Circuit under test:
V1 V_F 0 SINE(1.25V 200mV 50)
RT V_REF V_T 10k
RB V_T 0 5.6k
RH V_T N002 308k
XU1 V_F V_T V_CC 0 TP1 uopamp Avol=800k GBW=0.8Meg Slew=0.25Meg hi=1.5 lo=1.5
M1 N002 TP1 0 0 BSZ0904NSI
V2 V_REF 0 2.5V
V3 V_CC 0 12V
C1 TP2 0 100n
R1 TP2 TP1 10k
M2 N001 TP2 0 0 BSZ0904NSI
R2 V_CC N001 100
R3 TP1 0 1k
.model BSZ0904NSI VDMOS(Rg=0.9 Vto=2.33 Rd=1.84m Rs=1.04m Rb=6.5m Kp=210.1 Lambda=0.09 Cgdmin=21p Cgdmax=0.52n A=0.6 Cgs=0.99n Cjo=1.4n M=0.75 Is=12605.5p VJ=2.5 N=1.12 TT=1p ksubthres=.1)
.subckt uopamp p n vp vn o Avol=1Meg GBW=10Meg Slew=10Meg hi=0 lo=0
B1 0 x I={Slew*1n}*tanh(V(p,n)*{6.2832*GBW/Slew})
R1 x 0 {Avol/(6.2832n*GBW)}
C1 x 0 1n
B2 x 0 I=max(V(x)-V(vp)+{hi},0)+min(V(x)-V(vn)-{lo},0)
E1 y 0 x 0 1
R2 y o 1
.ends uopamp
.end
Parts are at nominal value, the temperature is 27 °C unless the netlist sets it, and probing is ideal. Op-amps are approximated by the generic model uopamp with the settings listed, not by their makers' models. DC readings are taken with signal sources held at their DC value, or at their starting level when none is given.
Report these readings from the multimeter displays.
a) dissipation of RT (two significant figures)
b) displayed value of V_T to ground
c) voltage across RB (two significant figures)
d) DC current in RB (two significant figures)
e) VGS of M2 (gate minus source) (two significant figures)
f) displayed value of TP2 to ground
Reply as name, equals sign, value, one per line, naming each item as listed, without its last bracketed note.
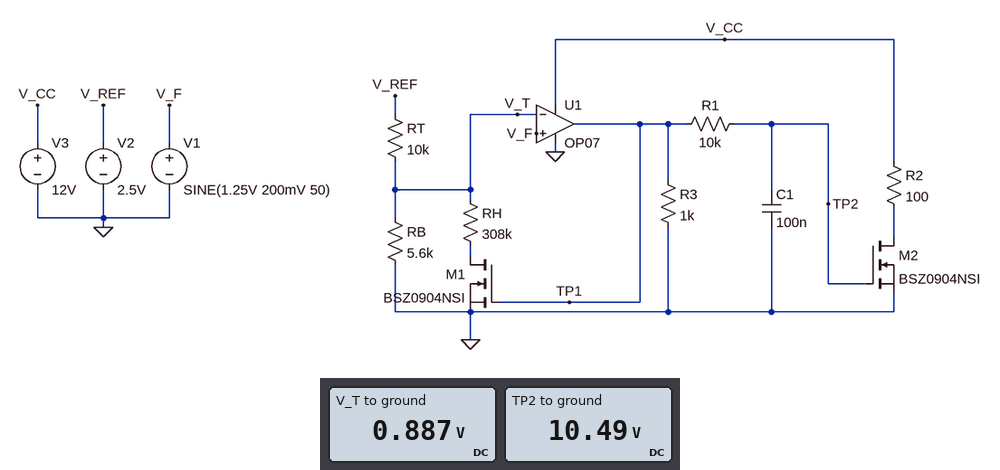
dissipation of RT = 260 µW
displayed value of V_T to ground = 0.887 V
voltage across RB = 890 mV
DC current in RB = 160 µA
VGS of M2 (gate minus source) = 10 V
displayed value of TP2 to ground = 10.49 V
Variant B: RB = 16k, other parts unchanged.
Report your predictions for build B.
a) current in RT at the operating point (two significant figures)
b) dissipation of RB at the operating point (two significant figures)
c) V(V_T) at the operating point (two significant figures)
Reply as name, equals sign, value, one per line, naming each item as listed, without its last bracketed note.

current in RT at the operating point = 96 µA
dissipation of RB at the operating point = 150 µW
V(V_T) at the operating point = 1.5 V
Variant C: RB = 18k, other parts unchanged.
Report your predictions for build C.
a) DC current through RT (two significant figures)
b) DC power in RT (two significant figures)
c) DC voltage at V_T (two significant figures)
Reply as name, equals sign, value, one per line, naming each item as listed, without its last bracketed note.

DC current through RT = 89 µA
DC power in RT = 80 µW
DC voltage at V_T = 1.6 V
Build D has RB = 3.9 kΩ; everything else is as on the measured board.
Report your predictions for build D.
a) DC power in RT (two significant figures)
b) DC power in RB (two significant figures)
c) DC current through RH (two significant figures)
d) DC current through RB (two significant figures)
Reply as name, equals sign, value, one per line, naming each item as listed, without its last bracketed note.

DC power in RT = 330 µW
DC power in RB = 120 µW
DC current through RH = 2.3 µA
DC current through RB = 180 µA
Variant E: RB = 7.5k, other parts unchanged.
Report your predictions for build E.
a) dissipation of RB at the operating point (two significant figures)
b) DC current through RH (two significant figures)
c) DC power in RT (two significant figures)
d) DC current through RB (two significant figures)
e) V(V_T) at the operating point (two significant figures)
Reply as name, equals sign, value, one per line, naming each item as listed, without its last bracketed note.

dissipation of RB at the operating point = 150 µW
DC current through RH = 3.4 µA
DC power in RT = 210 µW
DC current through RB = 140 µA
V(V_T) at the operating point = 1.1 V
